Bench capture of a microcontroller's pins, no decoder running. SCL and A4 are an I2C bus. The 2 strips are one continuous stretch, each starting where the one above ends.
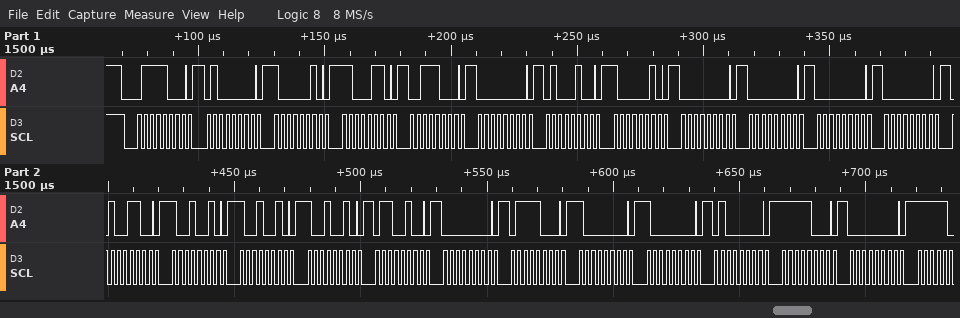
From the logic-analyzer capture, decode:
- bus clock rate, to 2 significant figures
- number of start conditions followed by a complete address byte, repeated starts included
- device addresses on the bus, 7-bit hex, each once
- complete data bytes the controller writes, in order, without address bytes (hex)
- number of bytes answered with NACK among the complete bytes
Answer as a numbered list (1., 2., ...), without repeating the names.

1. 400 kHz
2. 1
3. 0x3C
4. 40 82 C6 38 00 44 82 00 00 00 00 4C 92 92 92 64 00 78 80 80 40 F8 00
5. 0
